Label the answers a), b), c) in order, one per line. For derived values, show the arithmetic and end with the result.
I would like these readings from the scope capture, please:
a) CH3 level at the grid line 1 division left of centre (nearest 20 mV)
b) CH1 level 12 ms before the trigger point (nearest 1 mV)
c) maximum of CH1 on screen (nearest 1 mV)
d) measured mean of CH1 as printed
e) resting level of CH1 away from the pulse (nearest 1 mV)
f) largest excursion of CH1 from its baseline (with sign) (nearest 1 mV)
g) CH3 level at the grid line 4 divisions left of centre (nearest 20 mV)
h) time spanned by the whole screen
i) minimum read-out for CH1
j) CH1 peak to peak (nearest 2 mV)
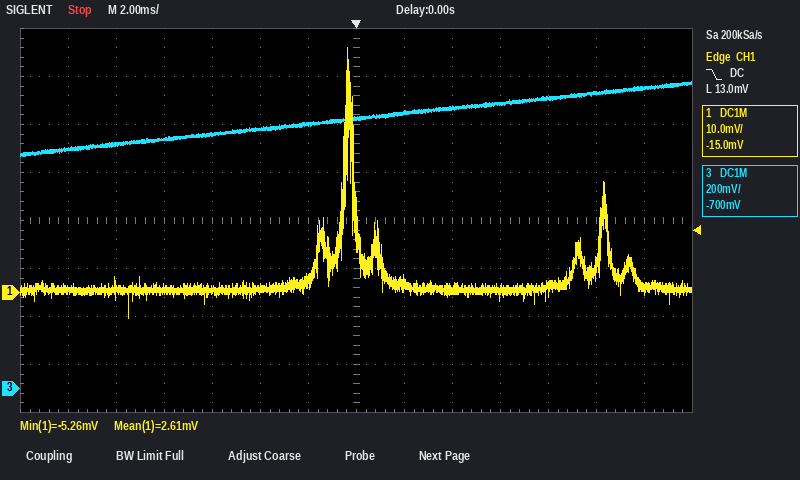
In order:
a) 1.10 V
b) 1 mV
c) 51 mV
d) 2.61 mV
e) 1 mV
f) 51 mV − (1 mV) = +50 mV
g) 1.04 V
h) 28 ms
i) -5.26 mV
j) 56 mV
